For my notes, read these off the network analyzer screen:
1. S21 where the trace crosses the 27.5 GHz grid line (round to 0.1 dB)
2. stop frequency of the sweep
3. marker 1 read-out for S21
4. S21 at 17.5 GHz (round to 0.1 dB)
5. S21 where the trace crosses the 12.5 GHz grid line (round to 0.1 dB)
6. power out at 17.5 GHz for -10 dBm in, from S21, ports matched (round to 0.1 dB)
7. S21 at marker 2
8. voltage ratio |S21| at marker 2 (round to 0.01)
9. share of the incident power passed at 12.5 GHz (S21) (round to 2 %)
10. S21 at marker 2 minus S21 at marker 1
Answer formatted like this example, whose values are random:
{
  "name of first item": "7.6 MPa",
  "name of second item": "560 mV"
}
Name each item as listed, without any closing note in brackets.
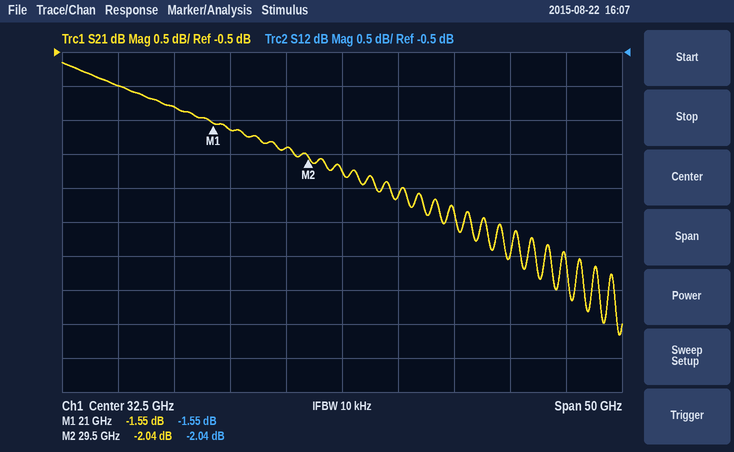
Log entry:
{
  "S21 where the trace crosses the 27.5 GHz grid line": "-1.9 dB",
  "stop frequency of the sweep": "57.5 GHz",
  "marker 1 read-out for S21": "-1.55 dB",
  "S21 at 17.5 GHz": "-1.3 dB",
  "S21 where the trace crosses the 12.5 GHz grid line": "-1.0 dB",
  "power out at 17.5 GHz for -10 dBm in, from S21, ports matched": "-11.3 dBm",
  "S21 at marker 2": "-2.04 dB",
  "voltage ratio |S21| at marker 2": "0.79",
  "share of the incident power passed at 12.5 GHz (S21)": "80 %",
  "S21 at marker 2 minus S21 at marker 1": "-0.49 dB"
}
